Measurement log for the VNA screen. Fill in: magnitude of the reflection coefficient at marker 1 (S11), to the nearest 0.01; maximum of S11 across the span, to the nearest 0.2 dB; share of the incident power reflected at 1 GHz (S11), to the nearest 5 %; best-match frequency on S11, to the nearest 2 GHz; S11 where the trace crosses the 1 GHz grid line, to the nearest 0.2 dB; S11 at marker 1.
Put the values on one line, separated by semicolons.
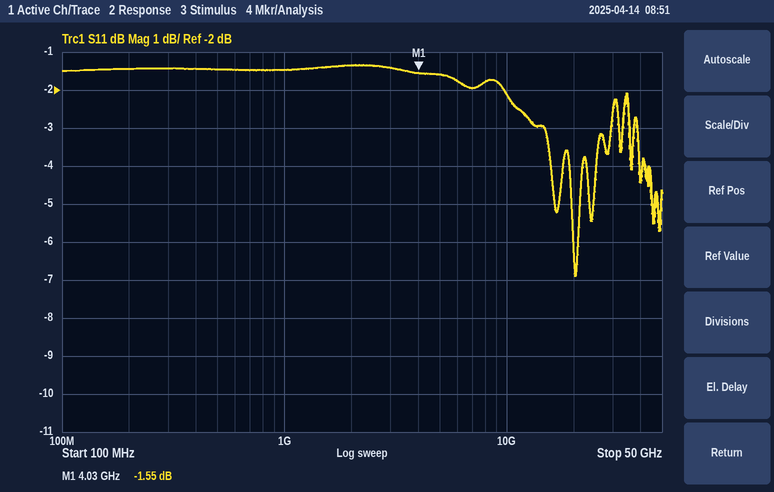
0.84; -1.4 dB; 70 %; 20 GHz; -1.4 dB; -1.55 dB
